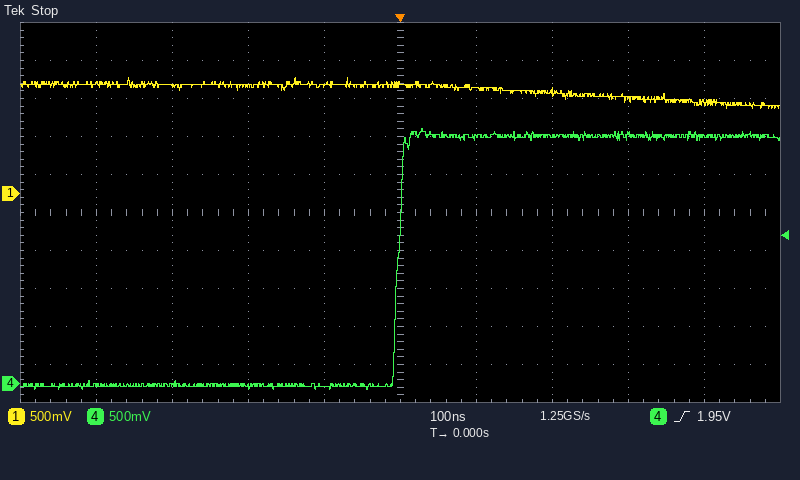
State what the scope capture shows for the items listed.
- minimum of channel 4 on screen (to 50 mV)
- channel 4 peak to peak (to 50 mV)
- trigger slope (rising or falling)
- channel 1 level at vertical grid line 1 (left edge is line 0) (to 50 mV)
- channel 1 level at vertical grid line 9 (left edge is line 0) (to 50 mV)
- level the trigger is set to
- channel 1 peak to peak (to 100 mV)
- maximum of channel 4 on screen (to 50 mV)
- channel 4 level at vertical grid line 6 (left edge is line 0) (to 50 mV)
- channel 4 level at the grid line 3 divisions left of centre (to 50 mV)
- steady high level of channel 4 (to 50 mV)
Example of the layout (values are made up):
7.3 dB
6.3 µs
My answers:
-100 mV
3.45 V
rising
1.45 V
1.20 V
1.95 V
400 mV
3.35 V
3.25 V
0 mV
3.25 V
